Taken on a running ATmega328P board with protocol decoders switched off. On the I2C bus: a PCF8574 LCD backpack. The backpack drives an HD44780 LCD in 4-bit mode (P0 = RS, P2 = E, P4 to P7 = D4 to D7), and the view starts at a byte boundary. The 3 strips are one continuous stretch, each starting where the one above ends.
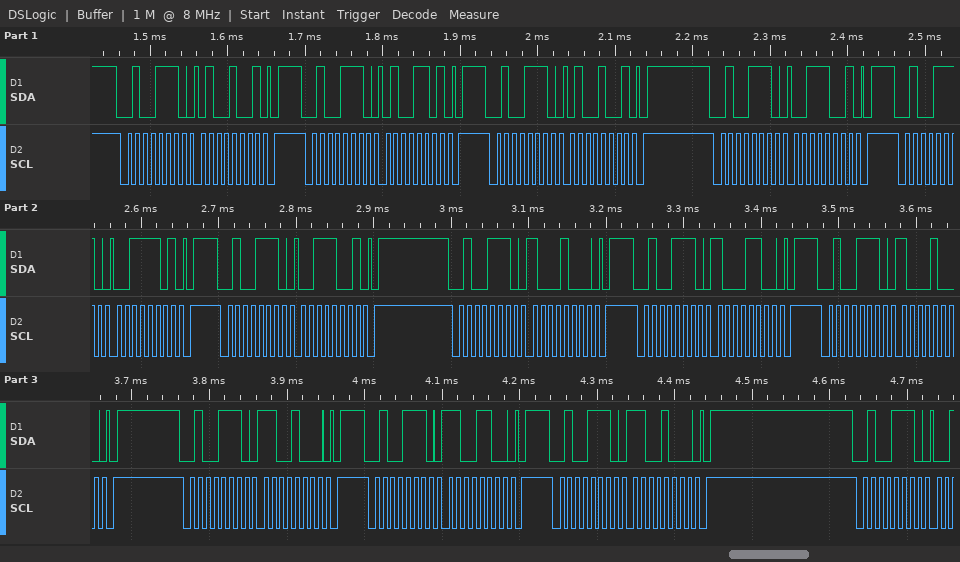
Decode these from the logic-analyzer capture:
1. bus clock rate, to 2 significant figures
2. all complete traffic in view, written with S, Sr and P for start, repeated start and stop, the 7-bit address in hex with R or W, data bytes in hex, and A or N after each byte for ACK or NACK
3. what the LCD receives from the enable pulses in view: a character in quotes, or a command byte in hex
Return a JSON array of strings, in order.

["100 kHz", "S 27W A 49 A P S 27W A 4D A P S 27W A 49 A P S 27W A 39 A P S 27W A 3D A P S 27W A 39 A P S 27W A 88 A P S 27W A 8C A P S 27W A 88 A P S 27W A C8 A P S 27W A CC A P S 27W A C8 A P S 27W A", "'C' 0x8C"]
